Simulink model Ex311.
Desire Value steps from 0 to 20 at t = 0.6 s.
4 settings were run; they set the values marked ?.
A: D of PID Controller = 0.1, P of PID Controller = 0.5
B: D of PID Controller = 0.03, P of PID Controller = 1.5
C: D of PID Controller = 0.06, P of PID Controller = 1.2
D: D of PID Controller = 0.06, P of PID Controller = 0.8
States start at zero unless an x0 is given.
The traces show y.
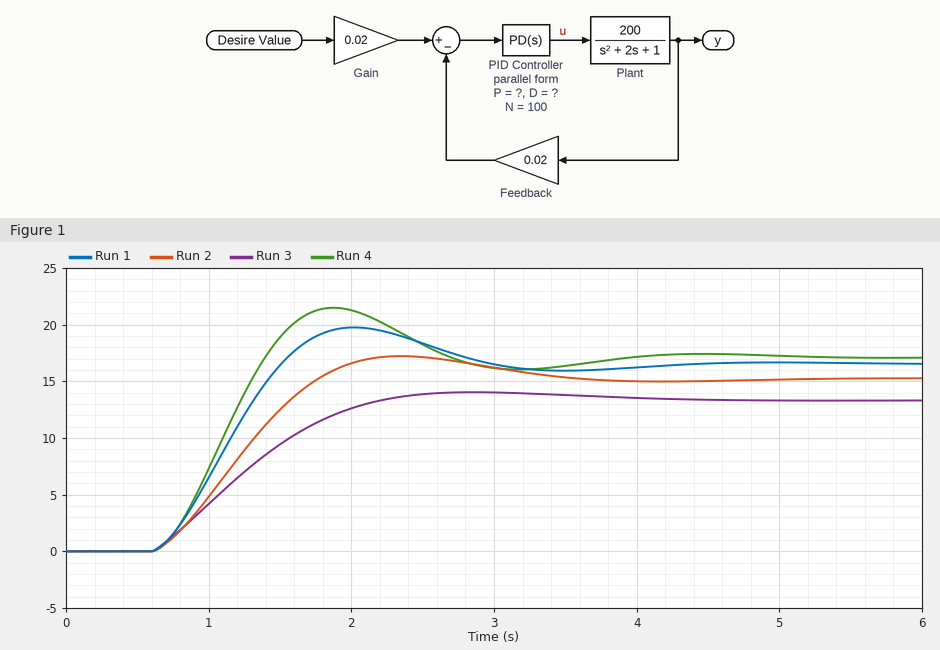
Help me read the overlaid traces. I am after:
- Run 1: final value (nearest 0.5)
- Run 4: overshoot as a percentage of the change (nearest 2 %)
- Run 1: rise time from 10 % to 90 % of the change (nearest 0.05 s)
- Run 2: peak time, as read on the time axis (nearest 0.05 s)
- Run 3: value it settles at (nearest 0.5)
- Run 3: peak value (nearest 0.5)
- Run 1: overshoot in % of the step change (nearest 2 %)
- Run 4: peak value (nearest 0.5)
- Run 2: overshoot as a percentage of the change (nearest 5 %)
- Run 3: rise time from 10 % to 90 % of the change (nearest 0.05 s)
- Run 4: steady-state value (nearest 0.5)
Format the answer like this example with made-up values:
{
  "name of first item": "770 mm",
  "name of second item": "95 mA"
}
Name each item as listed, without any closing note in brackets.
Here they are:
{
  "Run 1: final value": "16.5",
  "Run 4: overshoot as a percentage of the change": "26 %",
  "Run 1: rise time from 10 % to 90 % of the change": "0.65 s",
  "Run 2: peak time, as read on the time axis": "2.35 s",
  "Run 3: value it settles at": "13.5",
  "Run 3: peak value": "14.0",
  "Run 1: overshoot in % of the step change": "20 %",
  "Run 4: peak value": "21.5",
  "Run 2: overshoot as a percentage of the change": "15 %",
  "Run 3: rise time from 10 % to 90 % of the change": "1.10 s",
  "Run 4: steady-state value": "17.0"
}
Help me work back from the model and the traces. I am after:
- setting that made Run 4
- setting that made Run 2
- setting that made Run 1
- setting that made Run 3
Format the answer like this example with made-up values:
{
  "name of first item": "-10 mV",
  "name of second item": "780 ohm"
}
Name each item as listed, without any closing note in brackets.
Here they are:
{
  "setting that made Run 4": "B",
  "setting that made Run 2": "D",
  "setting that made Run 1": "C",
  "setting that made Run 3": "A"
}
